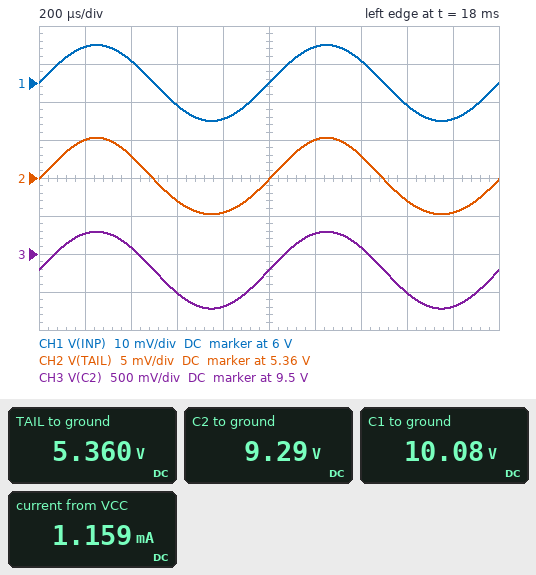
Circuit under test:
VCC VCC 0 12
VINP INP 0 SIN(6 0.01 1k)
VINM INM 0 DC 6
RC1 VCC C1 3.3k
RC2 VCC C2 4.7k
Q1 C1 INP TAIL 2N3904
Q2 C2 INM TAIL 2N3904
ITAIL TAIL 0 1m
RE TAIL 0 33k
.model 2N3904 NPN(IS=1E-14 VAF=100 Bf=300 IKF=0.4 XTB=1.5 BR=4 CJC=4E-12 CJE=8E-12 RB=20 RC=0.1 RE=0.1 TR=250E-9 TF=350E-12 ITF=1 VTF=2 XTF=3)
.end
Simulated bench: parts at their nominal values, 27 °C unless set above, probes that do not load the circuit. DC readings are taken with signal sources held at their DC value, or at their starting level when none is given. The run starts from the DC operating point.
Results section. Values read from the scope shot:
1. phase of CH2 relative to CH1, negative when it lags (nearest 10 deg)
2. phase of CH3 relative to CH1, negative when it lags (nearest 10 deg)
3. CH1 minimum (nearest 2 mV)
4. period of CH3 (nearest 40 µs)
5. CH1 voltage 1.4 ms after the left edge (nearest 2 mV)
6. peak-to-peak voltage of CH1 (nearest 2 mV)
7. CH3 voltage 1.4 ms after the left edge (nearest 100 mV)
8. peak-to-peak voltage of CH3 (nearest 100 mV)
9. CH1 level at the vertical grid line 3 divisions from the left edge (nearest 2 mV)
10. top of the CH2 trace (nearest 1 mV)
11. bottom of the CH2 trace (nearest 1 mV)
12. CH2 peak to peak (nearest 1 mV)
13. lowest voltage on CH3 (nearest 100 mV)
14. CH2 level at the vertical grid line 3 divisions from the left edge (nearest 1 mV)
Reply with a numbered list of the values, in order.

1. 0 deg
2. 0 deg
3. 5.990 V
4. 1.00 ms
5. 6.006 V
6. 20 mV
7. 9.6 V
8. 1.0 V
9. 5.994 V
10. 5.365 V
11. 5.355 V
12. 10 mV
13. 8.8 V
14. 5.357 V
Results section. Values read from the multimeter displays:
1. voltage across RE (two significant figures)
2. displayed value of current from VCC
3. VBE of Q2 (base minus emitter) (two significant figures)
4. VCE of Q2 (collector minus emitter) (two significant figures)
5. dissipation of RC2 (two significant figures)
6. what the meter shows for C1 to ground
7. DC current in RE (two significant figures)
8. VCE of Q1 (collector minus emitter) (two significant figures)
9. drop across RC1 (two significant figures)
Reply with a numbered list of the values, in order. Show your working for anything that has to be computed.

1. 5.36 V = 5.4 V
2. 1.159 mA
3. 6 V - 5.36 V = 640 mV
4. 9.29 V - 5.36 V = 3.9 V
5. (12 V - 9.29 V)^2 / 4.7 kΩ = 1.6 mW
6. 10.08 V
7. (5.36 V) / 33 kΩ = 160 µA
8. 10.08 V - 5.36 V = 4.7 V
9. 12 V - 10.08 V = 1.9 V
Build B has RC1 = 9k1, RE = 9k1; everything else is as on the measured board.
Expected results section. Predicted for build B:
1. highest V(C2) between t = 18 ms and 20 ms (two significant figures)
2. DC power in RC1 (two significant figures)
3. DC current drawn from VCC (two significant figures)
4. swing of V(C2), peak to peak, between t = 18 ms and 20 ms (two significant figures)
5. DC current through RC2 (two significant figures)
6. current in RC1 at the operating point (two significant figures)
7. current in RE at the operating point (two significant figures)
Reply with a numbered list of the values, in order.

1. 8.3 V
2. 4.8 mW
3. 1.6 mA
4. 750 mV
5. 840 µA
6. 720 µA
7. 590 µA
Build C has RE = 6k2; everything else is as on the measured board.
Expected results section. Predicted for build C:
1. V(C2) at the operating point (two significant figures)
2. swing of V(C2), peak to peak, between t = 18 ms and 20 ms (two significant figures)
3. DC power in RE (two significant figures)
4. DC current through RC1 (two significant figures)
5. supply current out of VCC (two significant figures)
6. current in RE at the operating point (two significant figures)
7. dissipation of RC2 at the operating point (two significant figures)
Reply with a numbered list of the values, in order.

1. 7.7 V
2. 1.6 V
3. 4.6 mW
4. 930 µA
5. 1.9 mA
6. 860 µA
7. 4.0 mW
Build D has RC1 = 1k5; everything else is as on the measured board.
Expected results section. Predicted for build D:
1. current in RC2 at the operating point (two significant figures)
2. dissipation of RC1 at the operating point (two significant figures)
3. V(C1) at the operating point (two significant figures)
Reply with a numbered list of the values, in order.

1. 570 µA
2. 510 µW
3. 11 V
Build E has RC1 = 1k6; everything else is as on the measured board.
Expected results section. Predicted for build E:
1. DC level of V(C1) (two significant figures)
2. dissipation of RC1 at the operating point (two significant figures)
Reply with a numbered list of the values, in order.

1. 11 V
2. 550 µW
